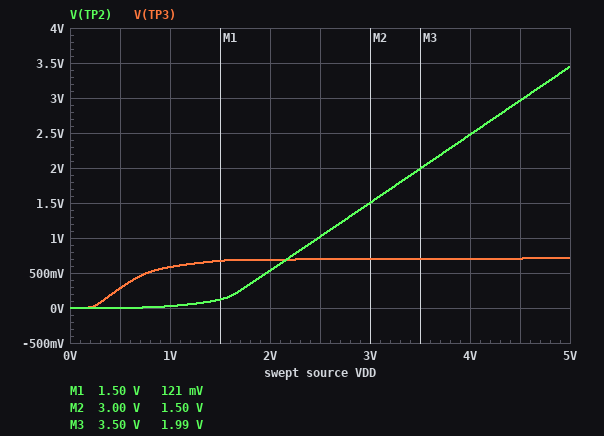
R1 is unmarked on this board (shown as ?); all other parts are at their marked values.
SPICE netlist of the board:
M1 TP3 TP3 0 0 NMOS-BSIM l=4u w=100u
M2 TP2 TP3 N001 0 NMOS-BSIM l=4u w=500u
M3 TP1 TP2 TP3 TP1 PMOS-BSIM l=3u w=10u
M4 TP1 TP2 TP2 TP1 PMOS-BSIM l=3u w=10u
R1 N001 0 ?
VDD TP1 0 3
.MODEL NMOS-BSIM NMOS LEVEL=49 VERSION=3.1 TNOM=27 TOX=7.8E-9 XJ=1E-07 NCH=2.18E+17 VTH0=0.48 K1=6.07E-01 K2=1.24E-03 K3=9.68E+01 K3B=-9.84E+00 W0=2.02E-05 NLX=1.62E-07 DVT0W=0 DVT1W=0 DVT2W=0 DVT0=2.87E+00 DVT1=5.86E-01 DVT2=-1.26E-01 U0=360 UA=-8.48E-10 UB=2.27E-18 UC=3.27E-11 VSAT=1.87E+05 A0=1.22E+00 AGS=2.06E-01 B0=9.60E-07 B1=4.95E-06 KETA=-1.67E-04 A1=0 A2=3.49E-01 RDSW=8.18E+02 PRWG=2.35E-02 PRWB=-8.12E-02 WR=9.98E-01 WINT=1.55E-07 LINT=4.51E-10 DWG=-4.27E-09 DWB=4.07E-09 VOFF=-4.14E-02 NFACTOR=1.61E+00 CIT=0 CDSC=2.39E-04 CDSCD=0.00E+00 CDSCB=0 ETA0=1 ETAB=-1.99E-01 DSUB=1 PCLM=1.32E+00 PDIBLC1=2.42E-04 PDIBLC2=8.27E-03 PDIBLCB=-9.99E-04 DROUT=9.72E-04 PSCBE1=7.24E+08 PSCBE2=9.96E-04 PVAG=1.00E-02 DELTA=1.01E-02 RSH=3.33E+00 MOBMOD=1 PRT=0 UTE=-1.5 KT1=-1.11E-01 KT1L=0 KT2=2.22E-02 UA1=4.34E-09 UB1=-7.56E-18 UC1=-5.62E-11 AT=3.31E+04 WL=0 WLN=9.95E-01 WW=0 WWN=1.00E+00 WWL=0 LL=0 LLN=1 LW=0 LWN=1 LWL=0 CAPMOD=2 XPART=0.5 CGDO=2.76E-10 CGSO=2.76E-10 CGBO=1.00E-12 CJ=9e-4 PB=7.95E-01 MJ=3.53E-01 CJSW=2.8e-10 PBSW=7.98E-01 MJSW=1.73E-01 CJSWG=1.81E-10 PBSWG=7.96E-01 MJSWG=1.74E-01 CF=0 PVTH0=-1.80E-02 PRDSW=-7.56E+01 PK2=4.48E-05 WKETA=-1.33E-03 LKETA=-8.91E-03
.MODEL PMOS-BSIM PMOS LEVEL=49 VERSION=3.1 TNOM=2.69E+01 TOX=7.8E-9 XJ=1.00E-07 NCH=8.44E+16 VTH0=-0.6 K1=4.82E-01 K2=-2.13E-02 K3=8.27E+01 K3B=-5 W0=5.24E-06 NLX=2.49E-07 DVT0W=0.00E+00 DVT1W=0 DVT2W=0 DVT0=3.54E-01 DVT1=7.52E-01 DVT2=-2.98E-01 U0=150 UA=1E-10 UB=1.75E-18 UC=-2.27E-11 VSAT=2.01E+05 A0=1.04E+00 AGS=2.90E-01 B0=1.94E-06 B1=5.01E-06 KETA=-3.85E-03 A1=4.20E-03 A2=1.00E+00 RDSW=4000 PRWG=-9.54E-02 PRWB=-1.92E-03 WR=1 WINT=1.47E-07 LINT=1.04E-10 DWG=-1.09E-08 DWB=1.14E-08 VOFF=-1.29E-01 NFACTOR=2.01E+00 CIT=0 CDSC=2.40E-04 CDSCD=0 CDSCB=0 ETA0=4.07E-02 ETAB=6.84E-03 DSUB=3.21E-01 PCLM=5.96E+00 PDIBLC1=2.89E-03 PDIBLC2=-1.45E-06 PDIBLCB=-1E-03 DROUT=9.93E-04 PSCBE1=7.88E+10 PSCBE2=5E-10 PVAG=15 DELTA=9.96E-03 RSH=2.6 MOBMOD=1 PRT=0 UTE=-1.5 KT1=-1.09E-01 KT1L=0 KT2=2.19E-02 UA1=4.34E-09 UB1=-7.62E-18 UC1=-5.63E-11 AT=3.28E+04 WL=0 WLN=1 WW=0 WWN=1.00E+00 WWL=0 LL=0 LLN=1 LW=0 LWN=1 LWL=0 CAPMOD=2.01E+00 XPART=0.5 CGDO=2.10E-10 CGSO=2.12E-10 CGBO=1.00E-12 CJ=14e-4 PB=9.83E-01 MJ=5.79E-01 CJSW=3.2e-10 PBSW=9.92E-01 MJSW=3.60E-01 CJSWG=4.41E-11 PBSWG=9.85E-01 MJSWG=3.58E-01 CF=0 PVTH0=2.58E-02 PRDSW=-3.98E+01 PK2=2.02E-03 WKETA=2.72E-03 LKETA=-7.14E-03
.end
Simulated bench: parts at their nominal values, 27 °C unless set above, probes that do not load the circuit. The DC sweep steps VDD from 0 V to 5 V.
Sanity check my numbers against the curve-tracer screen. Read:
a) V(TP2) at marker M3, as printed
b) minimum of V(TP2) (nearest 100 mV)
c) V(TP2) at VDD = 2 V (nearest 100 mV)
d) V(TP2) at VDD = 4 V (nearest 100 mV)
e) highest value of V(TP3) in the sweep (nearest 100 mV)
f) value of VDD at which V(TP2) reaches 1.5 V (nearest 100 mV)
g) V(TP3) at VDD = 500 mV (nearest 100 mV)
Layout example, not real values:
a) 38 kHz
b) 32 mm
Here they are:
a) 1.99 V
b) 0 V
c) 500 mV
d) 2.5 V
e) 700 mV
f) 3.0 V
g) 300 mV
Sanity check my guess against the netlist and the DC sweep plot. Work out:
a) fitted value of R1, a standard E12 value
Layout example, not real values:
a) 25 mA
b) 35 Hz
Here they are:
a) 1.5 kΩ
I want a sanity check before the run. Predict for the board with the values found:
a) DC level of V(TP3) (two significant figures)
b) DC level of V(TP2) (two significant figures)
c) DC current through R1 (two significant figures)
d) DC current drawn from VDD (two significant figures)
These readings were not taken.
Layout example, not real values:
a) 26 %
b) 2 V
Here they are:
a) 700 mV
b) 1.5 V
c) 56 µA
d) 110 µA
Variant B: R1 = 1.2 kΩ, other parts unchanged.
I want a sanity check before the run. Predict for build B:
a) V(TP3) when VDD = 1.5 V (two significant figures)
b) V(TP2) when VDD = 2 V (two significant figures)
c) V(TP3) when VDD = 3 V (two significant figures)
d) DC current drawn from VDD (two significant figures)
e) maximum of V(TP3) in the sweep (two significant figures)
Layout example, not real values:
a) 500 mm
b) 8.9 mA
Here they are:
a) 680 mV
b) 390 mV
c) 720 mV
d) 150 µA
e) 740 mV
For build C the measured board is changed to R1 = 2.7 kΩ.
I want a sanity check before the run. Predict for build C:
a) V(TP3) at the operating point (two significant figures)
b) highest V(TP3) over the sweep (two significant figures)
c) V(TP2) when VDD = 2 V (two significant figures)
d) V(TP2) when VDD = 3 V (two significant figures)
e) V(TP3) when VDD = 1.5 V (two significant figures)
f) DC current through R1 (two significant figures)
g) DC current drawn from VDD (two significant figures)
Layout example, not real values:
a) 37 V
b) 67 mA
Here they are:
a) 650 mV
b) 660 mV
c) 800 mV
d) 1.8 V
e) 640 mV
f) 27 µA
g) 55 µA
